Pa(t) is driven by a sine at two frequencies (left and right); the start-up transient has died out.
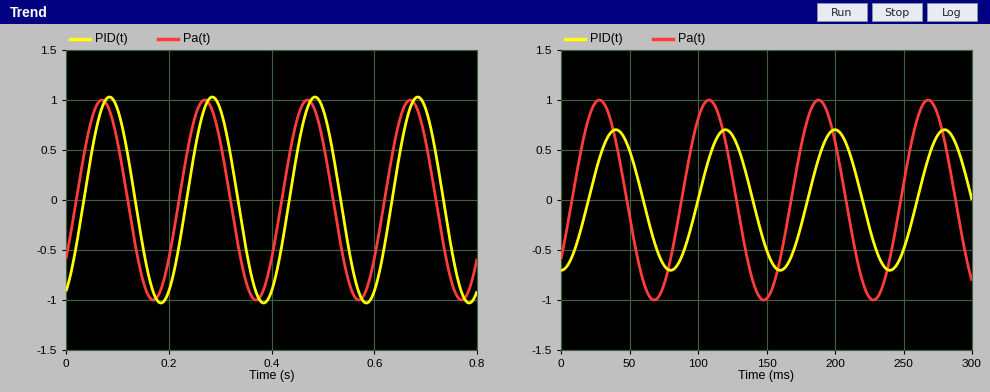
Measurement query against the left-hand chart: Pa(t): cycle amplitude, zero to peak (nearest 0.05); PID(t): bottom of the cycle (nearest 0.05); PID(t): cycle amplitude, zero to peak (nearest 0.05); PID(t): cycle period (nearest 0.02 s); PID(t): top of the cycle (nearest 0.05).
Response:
1.00
-1.05
1.05
0.20 s
1.05
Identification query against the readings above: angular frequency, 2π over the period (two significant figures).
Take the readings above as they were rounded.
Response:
31 rad/s
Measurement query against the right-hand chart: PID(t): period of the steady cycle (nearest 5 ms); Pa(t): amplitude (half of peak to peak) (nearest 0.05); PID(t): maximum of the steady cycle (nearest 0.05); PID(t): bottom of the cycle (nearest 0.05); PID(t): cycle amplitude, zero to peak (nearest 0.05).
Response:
80 ms
1.00
0.70
-0.70
0.70
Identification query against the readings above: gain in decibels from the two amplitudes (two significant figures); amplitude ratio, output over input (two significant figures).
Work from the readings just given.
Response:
-3.1 dB
0.70
